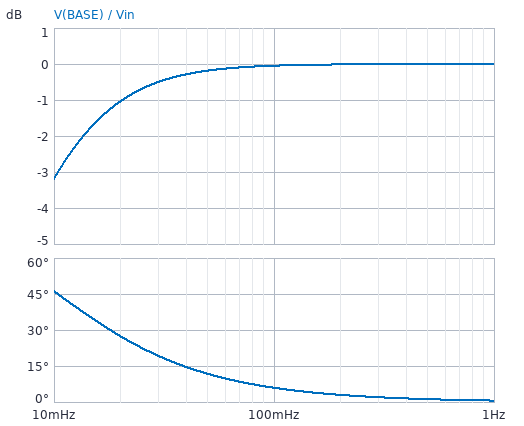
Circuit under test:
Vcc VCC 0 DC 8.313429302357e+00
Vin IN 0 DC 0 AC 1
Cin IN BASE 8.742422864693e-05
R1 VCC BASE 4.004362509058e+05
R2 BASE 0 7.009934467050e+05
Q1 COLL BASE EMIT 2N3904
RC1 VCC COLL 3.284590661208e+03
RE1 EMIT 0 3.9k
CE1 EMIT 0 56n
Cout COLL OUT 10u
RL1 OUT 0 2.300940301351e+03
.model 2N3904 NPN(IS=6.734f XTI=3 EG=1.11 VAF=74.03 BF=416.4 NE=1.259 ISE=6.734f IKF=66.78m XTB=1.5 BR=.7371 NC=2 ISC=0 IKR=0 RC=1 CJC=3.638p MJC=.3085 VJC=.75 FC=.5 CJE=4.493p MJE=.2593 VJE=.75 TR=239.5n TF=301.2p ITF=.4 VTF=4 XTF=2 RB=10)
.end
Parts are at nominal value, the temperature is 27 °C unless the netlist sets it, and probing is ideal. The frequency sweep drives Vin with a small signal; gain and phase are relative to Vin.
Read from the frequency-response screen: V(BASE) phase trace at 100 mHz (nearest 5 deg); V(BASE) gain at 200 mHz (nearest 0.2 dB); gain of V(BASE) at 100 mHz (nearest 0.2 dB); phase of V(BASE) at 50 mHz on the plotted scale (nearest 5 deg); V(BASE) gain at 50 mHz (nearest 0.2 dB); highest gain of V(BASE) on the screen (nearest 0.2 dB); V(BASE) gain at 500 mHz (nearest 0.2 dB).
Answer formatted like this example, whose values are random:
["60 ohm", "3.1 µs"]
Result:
["5 deg", "0 dB", "0 dB", "10 deg", "-0.2 dB", "0 dB", "0 dB"]
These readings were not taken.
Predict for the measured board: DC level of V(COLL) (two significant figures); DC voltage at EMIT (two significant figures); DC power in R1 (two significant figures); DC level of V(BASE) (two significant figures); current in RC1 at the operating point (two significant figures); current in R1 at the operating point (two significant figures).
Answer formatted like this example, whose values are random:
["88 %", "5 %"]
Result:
["5.7 V", "3.1 V", "52 µW", "3.8 V", "790 µA", "11 µA"]
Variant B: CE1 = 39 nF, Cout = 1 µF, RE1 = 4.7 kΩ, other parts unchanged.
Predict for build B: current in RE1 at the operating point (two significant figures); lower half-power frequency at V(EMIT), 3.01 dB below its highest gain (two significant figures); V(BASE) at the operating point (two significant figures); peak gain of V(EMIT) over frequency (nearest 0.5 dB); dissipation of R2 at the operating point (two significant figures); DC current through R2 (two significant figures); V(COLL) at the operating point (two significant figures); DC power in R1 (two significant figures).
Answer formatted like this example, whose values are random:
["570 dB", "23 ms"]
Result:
["700 µA", "9.9 mHz", "3.9 V", "0 dB", "22 µW", "5.6 µA", "6.0 V", "48 µW"]
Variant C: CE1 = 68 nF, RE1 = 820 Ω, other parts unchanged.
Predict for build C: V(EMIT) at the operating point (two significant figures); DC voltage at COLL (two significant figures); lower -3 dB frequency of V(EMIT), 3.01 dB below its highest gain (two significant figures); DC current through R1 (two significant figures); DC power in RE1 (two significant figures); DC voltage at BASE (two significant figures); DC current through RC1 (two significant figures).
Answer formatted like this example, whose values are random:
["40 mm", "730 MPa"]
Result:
["1.5 V", "2.5 V", "22 mHz", "15 µA", "2.6 mW", "2.1 V", "1.8 mA"]
